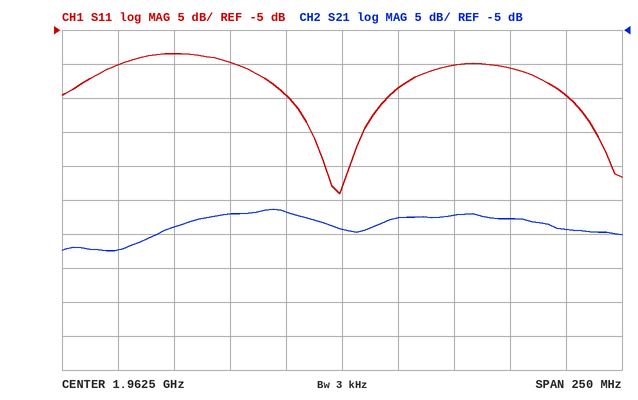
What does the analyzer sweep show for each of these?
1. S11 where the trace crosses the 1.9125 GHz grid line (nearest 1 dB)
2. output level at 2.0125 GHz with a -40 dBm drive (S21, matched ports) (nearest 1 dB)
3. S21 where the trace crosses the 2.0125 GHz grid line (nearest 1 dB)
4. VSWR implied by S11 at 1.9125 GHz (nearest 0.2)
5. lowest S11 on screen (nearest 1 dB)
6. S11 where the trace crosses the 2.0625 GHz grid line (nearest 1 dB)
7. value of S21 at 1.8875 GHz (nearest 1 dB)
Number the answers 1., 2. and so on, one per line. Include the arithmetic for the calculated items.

1. -10 dB
2. -40 dBm + (-32 dB) = -72 dBm
3. -32 dB
4. |Γ| = 10^(-10/20) = 0.3162; VSWR = (1 + 0.3162)/(1 − 0.3162) ≈ 1.92, so 2.0 to the nearest 0.2
5. -29 dB
6. -15 dB
7. -34 dB
